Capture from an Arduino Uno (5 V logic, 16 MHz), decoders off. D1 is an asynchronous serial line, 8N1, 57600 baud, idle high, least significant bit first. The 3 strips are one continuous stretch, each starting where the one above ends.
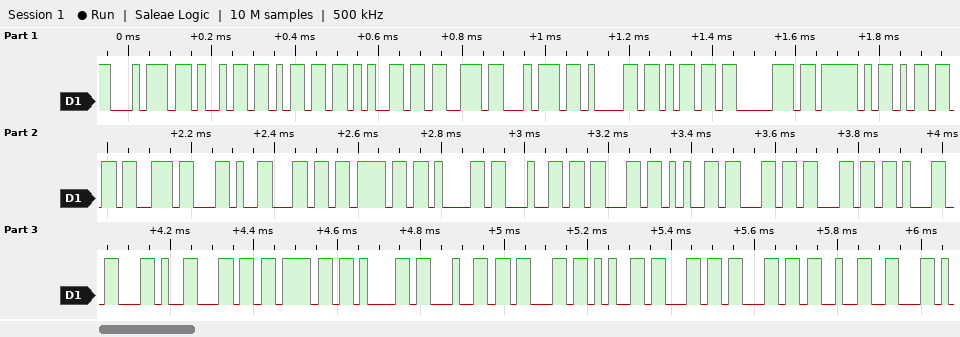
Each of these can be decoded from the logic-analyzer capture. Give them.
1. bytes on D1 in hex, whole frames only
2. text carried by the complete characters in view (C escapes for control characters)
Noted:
74 69 6D 65 73 74 61 6D 70 5F 6D 73 2C 6C 6F 61 64 63 65 6C 6C 31 2C 6C 6F 61 64 63 65 6C 6C 32
"timestamp_ms,loadcell1,loadcell2"
